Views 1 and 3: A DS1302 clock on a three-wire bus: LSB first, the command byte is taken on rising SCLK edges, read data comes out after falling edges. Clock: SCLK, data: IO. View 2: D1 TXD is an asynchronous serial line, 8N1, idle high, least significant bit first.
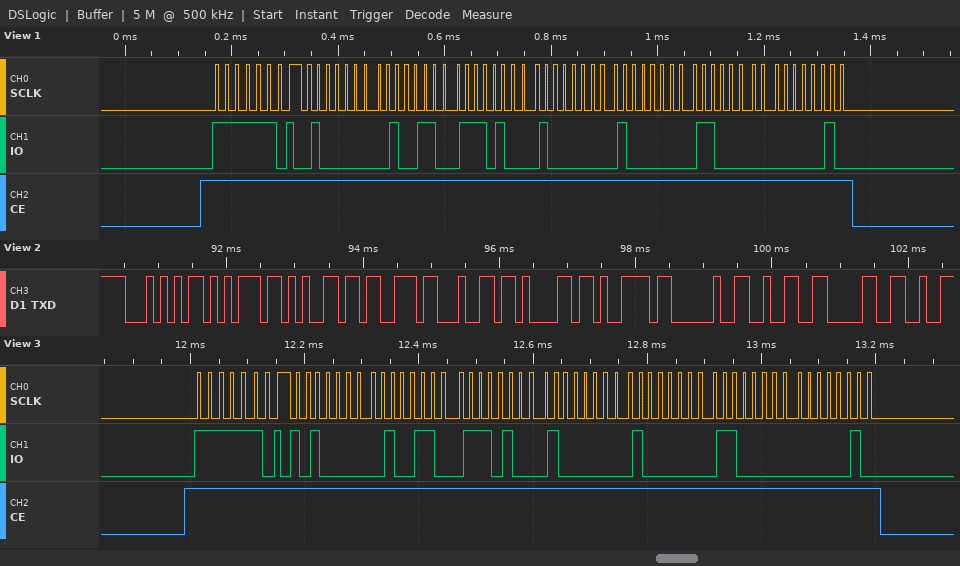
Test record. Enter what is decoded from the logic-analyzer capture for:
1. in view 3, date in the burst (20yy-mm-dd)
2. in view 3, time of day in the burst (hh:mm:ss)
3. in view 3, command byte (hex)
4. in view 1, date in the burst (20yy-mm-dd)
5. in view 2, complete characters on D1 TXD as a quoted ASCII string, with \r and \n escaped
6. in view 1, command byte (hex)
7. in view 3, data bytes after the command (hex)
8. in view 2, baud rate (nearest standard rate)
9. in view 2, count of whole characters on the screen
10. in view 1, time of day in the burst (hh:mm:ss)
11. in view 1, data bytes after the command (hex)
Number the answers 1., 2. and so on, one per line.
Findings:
1. 2020-01-01
2. 17:32:05
3. 0xBF
4. 2020-01-01
5. "Tuesday 20"
6. 0xBF
7. 05 32 17 01 01 03 20
8. 9600 baud
9. 10
10. 17:32:02
11. 02 32 17 01 01 03 20
